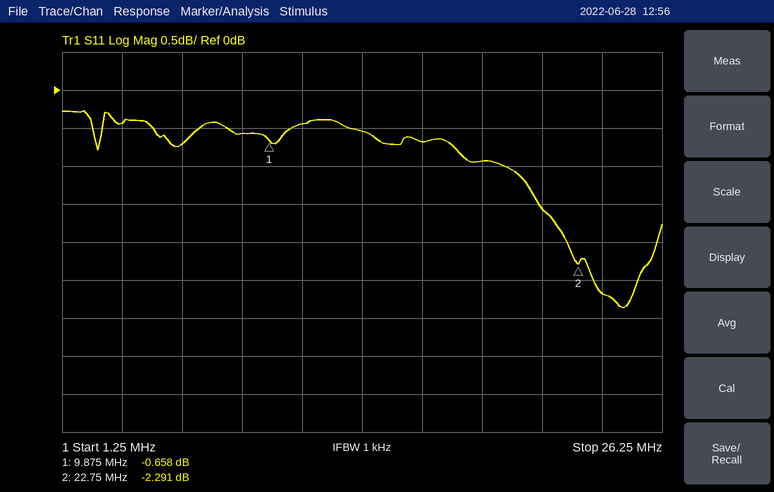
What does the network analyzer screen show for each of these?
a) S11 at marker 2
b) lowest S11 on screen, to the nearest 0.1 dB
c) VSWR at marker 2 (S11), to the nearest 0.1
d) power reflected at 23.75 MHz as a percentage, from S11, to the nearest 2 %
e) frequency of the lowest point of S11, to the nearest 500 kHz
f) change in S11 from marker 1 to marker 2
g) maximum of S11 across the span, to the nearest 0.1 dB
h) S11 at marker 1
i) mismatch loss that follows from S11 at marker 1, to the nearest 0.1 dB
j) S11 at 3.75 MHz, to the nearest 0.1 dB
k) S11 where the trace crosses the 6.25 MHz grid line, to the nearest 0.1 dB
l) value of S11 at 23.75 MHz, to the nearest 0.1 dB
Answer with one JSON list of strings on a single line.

["-2.291 dB", "-2.9 dB", "7.6", "54 %", "24.5 MHz", "-1.633 dB", "-0.3 dB", "-0.658 dB", "8.5 dB", "-0.4 dB", "-0.7 dB", "-2.7 dB"]
